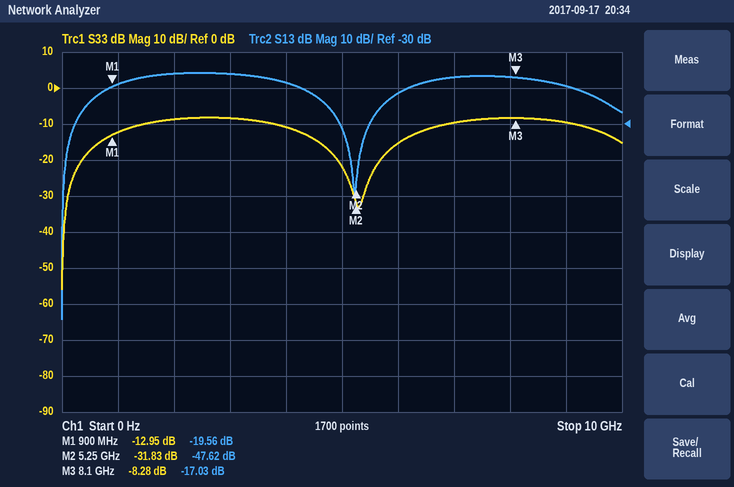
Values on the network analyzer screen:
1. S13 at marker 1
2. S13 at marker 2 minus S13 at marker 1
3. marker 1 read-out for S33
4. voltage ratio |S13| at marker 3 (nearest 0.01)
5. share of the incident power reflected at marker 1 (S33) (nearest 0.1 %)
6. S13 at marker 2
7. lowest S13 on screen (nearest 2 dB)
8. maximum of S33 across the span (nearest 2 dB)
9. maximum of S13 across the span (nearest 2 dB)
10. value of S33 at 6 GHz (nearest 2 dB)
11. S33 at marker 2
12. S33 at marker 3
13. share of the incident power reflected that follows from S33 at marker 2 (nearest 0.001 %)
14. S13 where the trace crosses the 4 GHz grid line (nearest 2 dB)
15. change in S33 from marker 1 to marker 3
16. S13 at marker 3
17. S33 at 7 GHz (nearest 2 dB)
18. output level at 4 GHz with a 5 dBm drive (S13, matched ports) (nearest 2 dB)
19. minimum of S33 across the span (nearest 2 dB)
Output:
-19.56 dB
-28.06 dB
-12.95 dB
0.14
5.1 %
-47.62 dB
-84 dB
-8 dB
-16 dB
-16 dB
-31.83 dB
-8.28 dB
0.066 %
-18 dB
4.67 dB
-17.03 dB
-10 dB
-14 dBm
-56 dB
